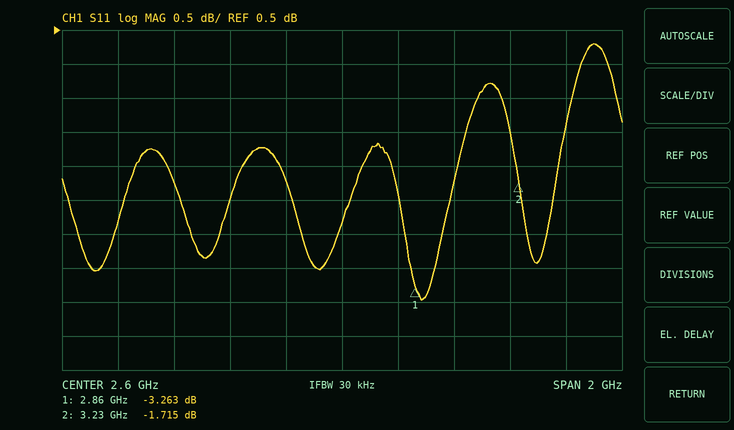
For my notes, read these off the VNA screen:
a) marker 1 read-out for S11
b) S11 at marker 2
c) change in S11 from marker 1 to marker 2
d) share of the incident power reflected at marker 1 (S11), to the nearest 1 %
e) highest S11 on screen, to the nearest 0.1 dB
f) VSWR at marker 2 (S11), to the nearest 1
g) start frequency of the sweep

-3.263 dB
-1.715 dB
1.548 dB
47 %
0.3 dB
10
1.6 GHz
